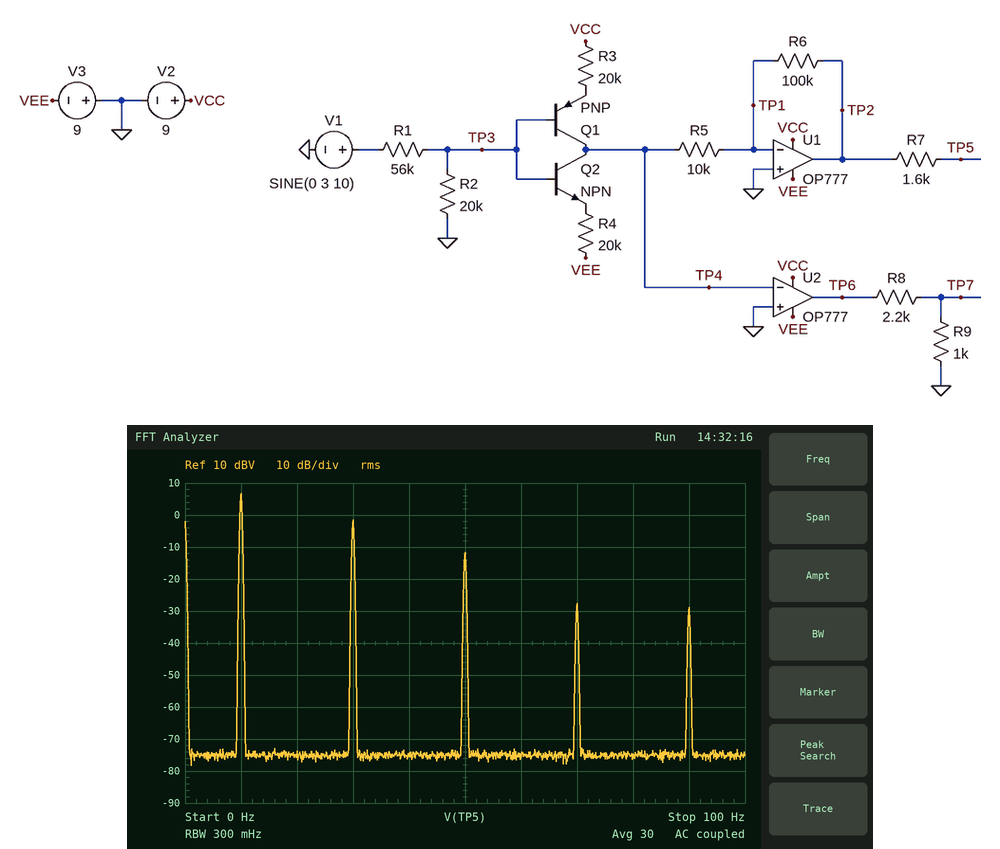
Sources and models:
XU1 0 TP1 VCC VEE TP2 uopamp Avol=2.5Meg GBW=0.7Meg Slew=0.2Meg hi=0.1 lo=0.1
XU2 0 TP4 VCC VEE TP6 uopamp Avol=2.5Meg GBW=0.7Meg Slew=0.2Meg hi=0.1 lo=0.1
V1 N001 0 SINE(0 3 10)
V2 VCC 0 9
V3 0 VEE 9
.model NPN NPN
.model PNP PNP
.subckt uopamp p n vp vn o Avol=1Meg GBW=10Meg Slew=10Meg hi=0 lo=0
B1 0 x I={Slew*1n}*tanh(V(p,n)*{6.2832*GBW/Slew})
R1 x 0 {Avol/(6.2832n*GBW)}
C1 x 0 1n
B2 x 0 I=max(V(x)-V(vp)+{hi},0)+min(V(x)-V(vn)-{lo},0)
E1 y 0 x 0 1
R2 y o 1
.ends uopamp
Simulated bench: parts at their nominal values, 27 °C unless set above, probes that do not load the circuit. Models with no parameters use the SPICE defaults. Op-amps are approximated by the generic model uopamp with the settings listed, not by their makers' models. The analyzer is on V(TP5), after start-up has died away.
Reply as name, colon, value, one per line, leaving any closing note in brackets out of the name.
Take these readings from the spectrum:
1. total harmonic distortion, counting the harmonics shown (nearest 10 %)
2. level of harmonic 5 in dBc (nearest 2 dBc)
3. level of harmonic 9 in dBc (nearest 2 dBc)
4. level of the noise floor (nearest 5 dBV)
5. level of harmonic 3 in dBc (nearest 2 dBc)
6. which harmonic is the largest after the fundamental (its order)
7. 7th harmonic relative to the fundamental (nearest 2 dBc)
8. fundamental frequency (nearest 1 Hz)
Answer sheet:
total harmonic distortion, counting the harmonics shown: 40 %
level of harmonic 5 in dBc: -18 dBc
level of harmonic 9 in dBc: -36 dBc
level of the noise floor: -75 dBV
level of harmonic 3 in dBc: -8 dBc
which harmonic is the largest after the fundamental: 3
7th harmonic relative to the fundamental: -34 dBc
fundamental frequency: 10 Hz
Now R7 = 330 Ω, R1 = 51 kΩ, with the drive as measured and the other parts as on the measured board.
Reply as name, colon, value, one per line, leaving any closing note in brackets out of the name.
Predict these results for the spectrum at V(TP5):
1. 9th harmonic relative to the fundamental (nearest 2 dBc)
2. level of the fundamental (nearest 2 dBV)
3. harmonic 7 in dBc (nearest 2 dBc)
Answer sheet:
9th harmonic relative to the fundamental: -40 dBc
level of the fundamental: 6 dBV
harmonic 7 in dBc: -30 dBc
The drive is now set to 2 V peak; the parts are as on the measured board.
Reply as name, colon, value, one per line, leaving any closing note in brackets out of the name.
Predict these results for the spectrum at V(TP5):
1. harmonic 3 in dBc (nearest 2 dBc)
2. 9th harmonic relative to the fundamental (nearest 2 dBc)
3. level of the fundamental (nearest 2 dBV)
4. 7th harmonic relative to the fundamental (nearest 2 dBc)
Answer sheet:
harmonic 3 in dBc: -14 dBc
9th harmonic relative to the fundamental: -40 dBc
level of the fundamental: 8 dBV
7th harmonic relative to the fundamental: -32 dBc
